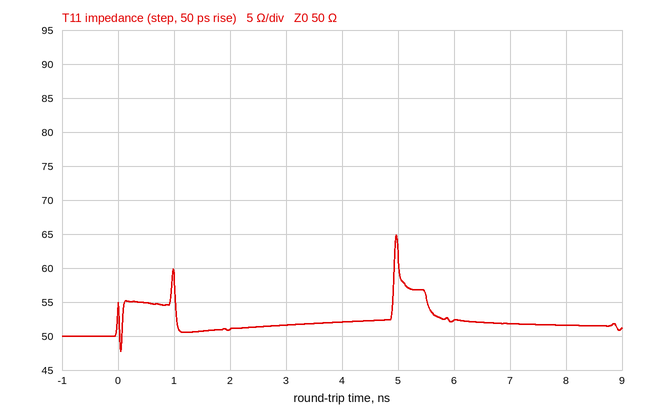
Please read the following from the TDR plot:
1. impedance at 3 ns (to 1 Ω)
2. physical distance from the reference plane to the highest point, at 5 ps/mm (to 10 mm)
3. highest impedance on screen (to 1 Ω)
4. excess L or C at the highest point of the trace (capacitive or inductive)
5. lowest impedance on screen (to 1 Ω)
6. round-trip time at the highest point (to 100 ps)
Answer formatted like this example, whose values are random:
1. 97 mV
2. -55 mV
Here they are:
1. 52 Ω
2. 500 mm
3. 65 Ω
4. inductive
5. 48 Ω
6. 5.0 ns
